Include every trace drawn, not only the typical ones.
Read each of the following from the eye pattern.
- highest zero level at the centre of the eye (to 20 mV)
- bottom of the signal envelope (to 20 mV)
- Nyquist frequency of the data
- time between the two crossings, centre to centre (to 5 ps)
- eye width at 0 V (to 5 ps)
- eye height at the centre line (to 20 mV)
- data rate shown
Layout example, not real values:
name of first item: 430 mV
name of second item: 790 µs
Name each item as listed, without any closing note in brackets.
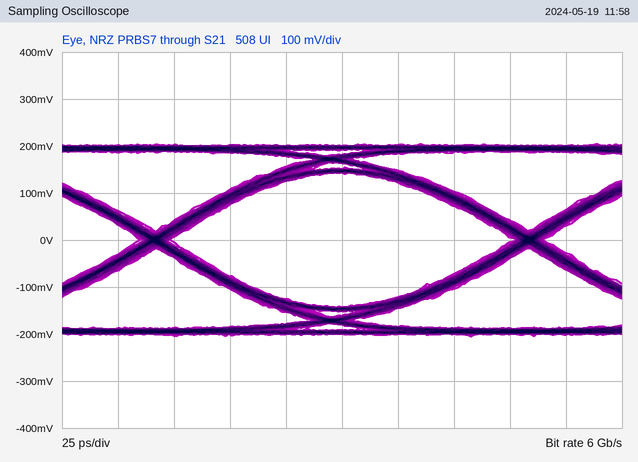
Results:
highest zero level at the centre of the eye: -140 mV
bottom of the signal envelope: -200 mV
Nyquist frequency of the data: 3 GHz
time between the two crossings, centre to centre: 165 ps
eye width at 0 V: 155 ps
eye height at the centre line: 280 mV
data rate shown: 6 Gb/s
